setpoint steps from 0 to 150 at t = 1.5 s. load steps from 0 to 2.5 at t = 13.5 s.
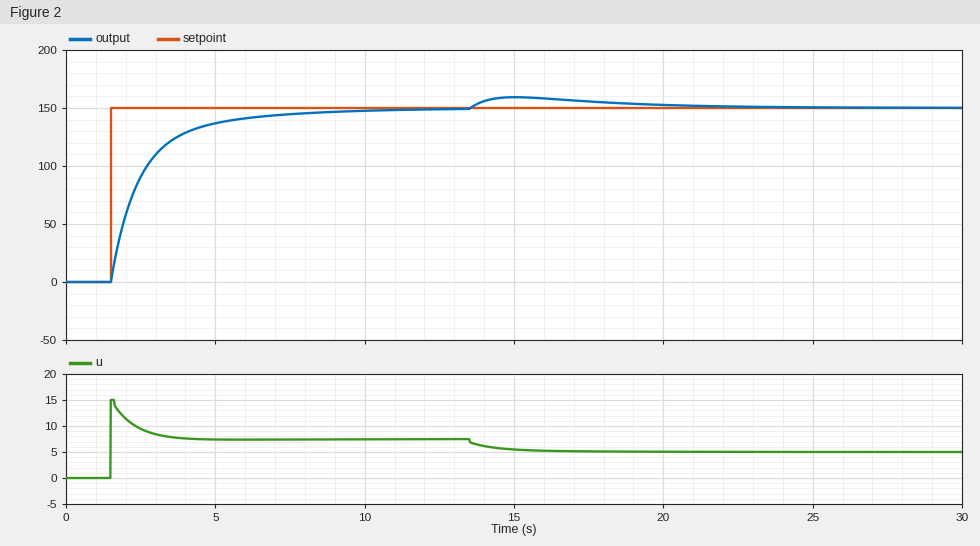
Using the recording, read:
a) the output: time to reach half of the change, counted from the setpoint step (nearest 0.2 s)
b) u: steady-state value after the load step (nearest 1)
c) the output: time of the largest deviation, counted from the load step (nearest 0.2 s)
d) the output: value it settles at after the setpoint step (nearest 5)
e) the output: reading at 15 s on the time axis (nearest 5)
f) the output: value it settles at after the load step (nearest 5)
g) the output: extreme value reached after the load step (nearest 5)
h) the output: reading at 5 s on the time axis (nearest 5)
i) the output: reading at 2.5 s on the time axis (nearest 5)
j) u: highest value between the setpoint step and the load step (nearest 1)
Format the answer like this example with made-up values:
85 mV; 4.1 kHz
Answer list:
0.8 s; 5; 1.6 s; 150; 160; 150; 160; 135; 90; 15
